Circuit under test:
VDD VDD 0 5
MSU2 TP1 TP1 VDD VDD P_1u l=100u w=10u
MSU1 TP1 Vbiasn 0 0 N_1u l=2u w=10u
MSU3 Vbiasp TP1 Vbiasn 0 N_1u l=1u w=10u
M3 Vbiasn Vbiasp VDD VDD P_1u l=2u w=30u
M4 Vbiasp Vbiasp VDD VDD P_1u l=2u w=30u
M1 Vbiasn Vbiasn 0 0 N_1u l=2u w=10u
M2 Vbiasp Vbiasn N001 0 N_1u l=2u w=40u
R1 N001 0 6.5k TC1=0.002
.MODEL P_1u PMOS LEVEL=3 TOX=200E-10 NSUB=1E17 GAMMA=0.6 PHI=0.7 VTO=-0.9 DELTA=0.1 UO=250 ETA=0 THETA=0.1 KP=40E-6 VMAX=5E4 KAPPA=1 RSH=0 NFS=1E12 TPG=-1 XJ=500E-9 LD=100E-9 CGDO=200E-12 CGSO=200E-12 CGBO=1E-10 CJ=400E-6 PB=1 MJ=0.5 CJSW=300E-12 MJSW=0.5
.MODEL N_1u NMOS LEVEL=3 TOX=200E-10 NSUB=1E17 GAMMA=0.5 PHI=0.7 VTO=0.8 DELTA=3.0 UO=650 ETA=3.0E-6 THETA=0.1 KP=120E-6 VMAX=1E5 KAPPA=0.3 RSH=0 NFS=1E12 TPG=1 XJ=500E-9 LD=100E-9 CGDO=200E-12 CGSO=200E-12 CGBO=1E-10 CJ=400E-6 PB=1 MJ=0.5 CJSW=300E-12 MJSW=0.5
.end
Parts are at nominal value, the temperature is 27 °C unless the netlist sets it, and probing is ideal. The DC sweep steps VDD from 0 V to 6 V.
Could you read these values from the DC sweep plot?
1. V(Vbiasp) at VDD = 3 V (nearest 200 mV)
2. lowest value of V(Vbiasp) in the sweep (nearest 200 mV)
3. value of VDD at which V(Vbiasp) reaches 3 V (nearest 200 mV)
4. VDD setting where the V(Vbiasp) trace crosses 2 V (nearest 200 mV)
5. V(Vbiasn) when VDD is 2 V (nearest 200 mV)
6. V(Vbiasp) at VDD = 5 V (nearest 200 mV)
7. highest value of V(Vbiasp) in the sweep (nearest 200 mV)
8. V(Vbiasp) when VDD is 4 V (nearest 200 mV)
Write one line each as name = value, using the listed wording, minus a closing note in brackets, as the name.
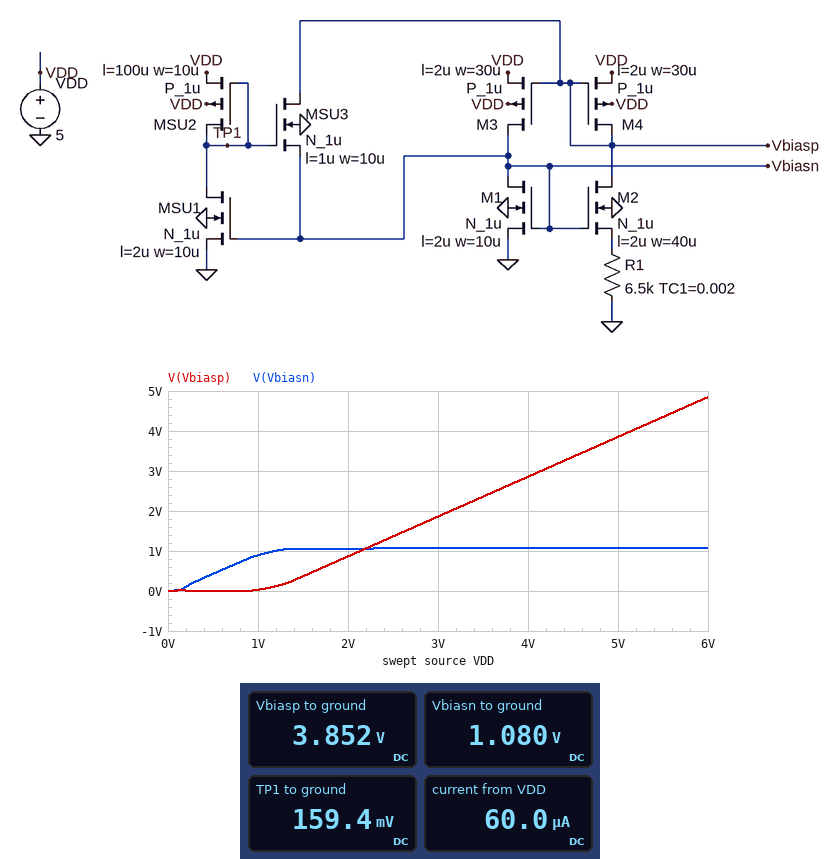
V(Vbiasp) at VDD = 3 V = 1.8 V
lowest value of V(Vbiasp) in the sweep = 0 V
value of VDD at which V(Vbiasp) reaches 3 V = 4.2 V
VDD setting where the V(Vbiasp) trace crosses 2 V = 3.2 V
V(Vbiasn) when VDD is 2 V = 1.0 V
V(Vbiasp) at VDD = 5 V = 3.8 V
highest value of V(Vbiasp) in the sweep = 4.8 V
V(Vbiasp) when VDD is 4 V = 2.8 V
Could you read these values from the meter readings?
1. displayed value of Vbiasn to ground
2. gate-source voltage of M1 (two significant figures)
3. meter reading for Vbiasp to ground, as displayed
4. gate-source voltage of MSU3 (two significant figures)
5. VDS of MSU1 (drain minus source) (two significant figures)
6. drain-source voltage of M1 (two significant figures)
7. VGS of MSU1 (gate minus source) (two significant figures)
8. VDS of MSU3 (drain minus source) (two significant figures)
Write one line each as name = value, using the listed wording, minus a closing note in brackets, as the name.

displayed value of Vbiasn to ground = 1.080 V
gate-source voltage of M1 = 1.1 V
meter reading for Vbiasp to ground, as displayed = 3.852 V
gate-source voltage of MSU3 = -920 mV
VDS of MSU1 (drain minus source) = 160 mV
drain-source voltage of M1 = 1.1 V
VGS of MSU1 (gate minus source) = 1.1 V
VDS of MSU3 (drain minus source) = 2.8 V
